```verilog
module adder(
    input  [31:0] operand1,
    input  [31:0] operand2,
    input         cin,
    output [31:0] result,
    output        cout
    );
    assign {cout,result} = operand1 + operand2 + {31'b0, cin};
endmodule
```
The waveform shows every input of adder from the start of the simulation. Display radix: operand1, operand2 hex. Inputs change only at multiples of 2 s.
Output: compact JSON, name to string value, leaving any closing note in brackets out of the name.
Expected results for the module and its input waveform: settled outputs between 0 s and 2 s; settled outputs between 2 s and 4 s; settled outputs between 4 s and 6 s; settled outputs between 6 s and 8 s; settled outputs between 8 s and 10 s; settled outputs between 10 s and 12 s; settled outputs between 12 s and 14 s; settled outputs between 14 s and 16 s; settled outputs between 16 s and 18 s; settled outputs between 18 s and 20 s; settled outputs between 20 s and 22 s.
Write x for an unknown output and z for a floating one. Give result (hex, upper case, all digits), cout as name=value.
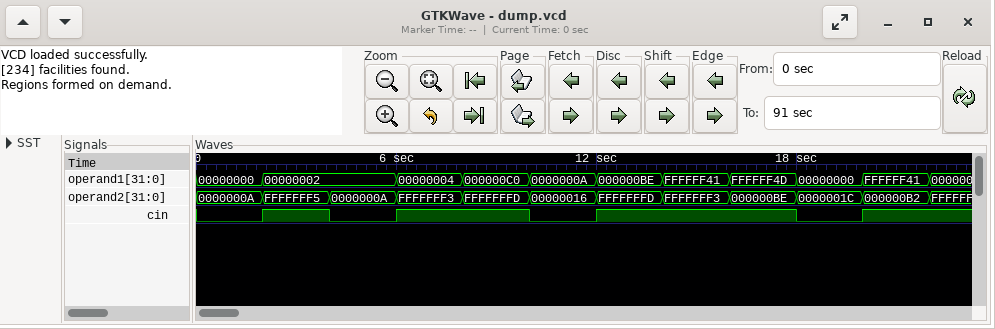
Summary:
{"settled outputs between 0 s and 2 s": "result=0000000A, cout=0", "settled outputs between 2 s and 4 s": "result=FFFFFFF8, cout=0", "settled outputs between 4 s and 6 s": "result=0000000C, cout=0", "settled outputs between 6 s and 8 s": "result=FFFFFFF8, cout=0", "settled outputs between 8 s and 10 s": "result=000000BE, cout=1", "settled outputs between 10 s and 12 s": "result=00000020, cout=0", "settled outputs between 12 s and 14 s": "result=000000BC, cout=1", "settled outputs between 14 s and 16 s": "result=FFFFFF35, cout=1", "settled outputs between 16 s and 18 s": "result=0000000C, cout=1", "settled outputs between 18 s and 20 s": "result=0000001C, cout=0", "settled outputs between 20 s and 22 s": "result=FFFFFFF4, cout=0"}
